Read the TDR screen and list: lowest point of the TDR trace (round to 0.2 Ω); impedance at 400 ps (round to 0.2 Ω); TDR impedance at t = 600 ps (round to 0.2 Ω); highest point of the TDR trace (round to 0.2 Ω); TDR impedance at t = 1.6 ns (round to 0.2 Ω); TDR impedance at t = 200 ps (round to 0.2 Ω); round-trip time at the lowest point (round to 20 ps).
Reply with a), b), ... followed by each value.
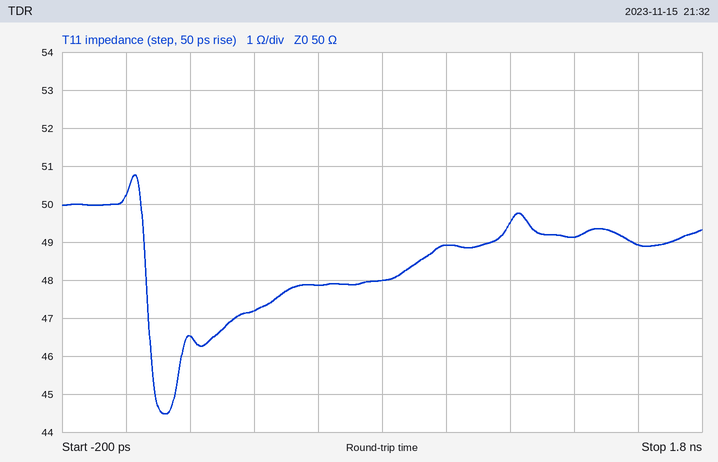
a) 44.4 Ω
b) 47.2 Ω
c) 47.8 Ω
d) 50.8 Ω
e) 49.0 Ω
f) 46.6 Ω
g) 120 ps
